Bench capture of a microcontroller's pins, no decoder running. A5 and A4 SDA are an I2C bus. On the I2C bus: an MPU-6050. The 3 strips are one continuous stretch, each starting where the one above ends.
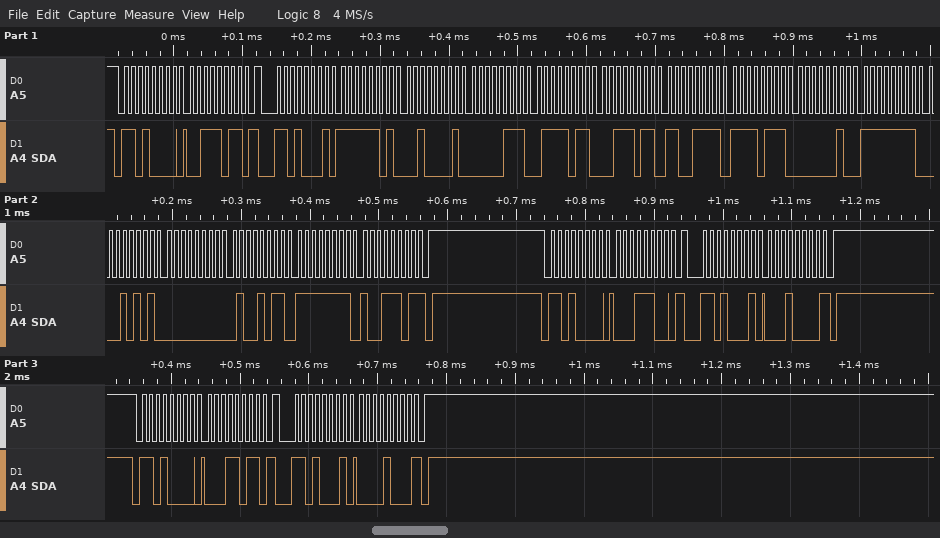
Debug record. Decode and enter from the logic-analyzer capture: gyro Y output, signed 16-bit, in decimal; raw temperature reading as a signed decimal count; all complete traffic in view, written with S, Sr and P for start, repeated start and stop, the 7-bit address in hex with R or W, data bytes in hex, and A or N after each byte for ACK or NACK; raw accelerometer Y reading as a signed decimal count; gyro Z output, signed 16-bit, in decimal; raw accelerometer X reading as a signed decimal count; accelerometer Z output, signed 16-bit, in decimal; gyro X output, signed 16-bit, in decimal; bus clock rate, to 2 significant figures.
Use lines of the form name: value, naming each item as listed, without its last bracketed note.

gyro Y output, signed 16-bit, in decimal: 75
raw temperature reading as a signed decimal count: -2302
all complete traffic in view, written with S, Sr and P for start, repeated start and stop, the 7-bit address in hex with R or W, data bytes in hex, and A or N after each byte for ACK or NACK: S 68W A 3B A Sr 68R A FD A 21 A 07 A 7B A 3B A CF A F7 A 02 A FF A 15 A 00 A 4B A FF A 9D N P S 68W A 1C A Sr 68R A 10 N P S 68W A 1B A Sr 68R A 08 N P
raw accelerometer Y reading as a signed decimal count: 1915
gyro Z output, signed 16-bit, in decimal: -99
raw accelerometer X reading as a signed decimal count: -735
accelerometer Z output, signed 16-bit, in decimal: 15311
gyro X output, signed 16-bit, in decimal: -235
bus clock rate, to 2 significant figures: 100 kHz
